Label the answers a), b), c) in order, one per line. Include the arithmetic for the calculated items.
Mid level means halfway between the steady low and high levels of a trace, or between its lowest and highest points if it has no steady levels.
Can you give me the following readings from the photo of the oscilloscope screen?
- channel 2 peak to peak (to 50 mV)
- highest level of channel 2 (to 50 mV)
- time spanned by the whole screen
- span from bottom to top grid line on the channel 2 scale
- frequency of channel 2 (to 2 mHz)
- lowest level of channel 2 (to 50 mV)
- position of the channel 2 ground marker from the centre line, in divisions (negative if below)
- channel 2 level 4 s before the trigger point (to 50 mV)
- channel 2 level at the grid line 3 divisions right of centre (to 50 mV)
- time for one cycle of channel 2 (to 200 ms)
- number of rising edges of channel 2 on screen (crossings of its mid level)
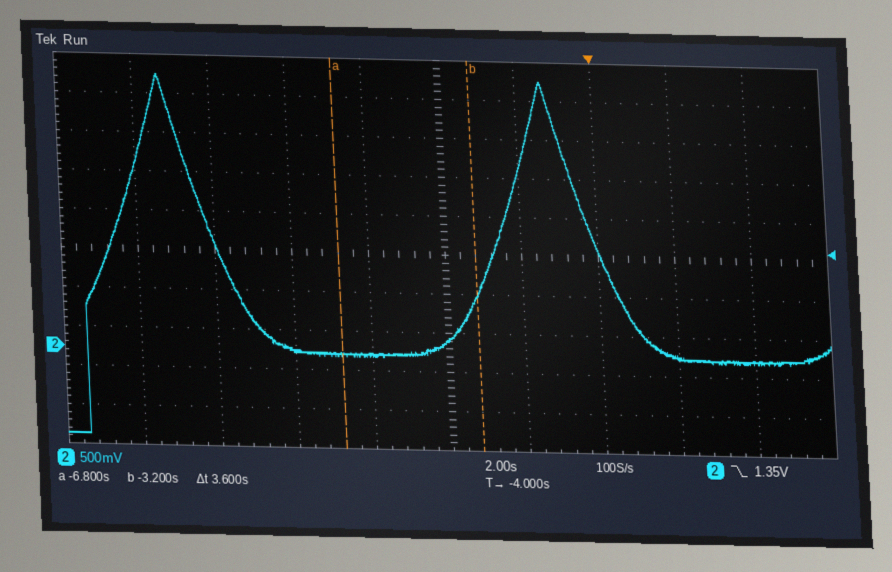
a) 3.50 V − (-1.10 V) = 4.60 V
b) 3.50 V
c) 20 s
d) 5 V
e) 1 / 10.0 s ≈ 100 mHz
f) -1.10 V
g) -2.5 div
h) 150 mV
i) 0 mV
j) 10.0 s
k) 2
